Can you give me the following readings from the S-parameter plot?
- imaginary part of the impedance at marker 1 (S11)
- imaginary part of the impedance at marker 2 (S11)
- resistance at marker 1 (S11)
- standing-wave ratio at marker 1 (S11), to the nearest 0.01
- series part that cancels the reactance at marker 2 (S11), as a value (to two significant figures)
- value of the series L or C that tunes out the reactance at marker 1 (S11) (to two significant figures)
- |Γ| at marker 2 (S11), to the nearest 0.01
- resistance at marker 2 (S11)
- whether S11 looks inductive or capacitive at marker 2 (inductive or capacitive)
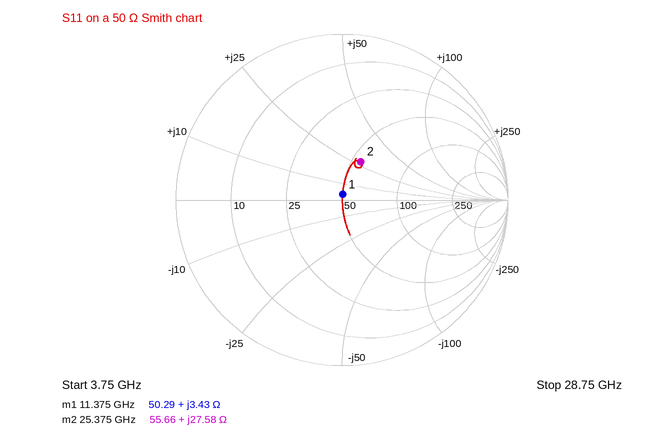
+3.43 Ω
+27.58 Ω
50.29 Ω
1.07
230 fF
4.1 pF
0.26
55.66 Ω
inductive
